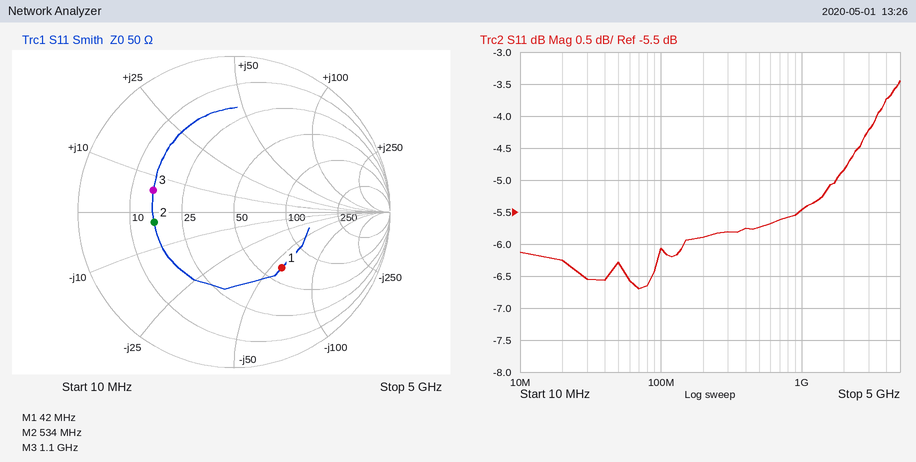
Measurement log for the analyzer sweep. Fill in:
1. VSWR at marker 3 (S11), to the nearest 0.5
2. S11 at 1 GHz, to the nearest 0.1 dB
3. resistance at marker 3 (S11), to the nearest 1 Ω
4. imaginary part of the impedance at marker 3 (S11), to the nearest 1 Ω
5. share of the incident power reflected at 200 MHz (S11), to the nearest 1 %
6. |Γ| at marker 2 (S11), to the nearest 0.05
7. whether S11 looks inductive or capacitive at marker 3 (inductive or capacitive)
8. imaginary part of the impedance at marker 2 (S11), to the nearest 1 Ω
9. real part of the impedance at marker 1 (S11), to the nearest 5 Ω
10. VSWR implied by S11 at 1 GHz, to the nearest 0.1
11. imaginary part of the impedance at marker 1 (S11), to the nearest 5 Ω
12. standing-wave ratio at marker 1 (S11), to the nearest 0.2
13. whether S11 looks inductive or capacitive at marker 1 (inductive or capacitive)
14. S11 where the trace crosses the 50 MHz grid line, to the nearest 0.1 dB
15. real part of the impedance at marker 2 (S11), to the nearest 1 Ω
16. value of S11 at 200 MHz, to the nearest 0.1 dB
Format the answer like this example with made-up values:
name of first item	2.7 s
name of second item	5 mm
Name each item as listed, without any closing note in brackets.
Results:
VSWR at marker 3 (S11), to the nearest 0.5	3.5
S11 at 1 GHz, to the nearest 0.1 dB	-5.5 dB
resistance at marker 3 (S11), to the nearest 1 Ω	15 Ω
imaginary part of the impedance at marker 3 (S11), to the nearest 1 Ω	+6 Ω
share of the incident power reflected at 200 MHz (S11), to the nearest 1 %	26 %
|Γ| at marker 2 (S11), to the nearest 0.05	0.50
whether S11 looks inductive or capacitive at marker 3	inductive
imaginary part of the impedance at marker 2 (S11), to the nearest 1 Ω	-3 Ω
real part of the impedance at marker 1 (S11), to the nearest 5 Ω	65 Ω
VSWR implied by S11 at 1 GHz, to the nearest 0.1	3.3
imaginary part of the impedance at marker 1 (S11), to the nearest 5 Ω	-60 Ω
standing-wave ratio at marker 1 (S11), to the nearest 0.2	2.8
whether S11 looks inductive or capacitive at marker 1	capacitive
S11 where the trace crosses the 50 MHz grid line, to the nearest 0.1 dB	-6.3 dB
real part of the impedance at marker 2 (S11), to the nearest 1 Ω	16 Ω
value of S11 at 200 MHz, to the nearest 0.1 dB	-5.9 dB
